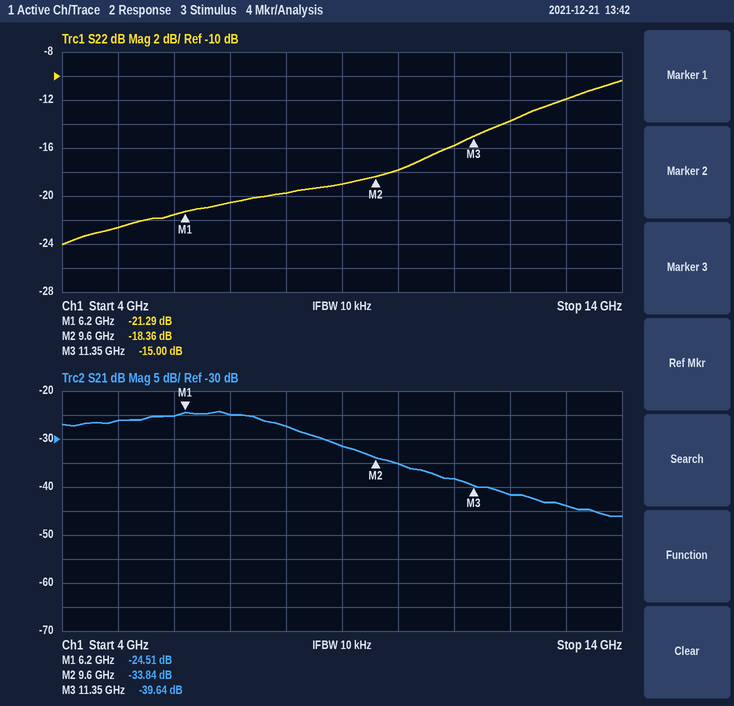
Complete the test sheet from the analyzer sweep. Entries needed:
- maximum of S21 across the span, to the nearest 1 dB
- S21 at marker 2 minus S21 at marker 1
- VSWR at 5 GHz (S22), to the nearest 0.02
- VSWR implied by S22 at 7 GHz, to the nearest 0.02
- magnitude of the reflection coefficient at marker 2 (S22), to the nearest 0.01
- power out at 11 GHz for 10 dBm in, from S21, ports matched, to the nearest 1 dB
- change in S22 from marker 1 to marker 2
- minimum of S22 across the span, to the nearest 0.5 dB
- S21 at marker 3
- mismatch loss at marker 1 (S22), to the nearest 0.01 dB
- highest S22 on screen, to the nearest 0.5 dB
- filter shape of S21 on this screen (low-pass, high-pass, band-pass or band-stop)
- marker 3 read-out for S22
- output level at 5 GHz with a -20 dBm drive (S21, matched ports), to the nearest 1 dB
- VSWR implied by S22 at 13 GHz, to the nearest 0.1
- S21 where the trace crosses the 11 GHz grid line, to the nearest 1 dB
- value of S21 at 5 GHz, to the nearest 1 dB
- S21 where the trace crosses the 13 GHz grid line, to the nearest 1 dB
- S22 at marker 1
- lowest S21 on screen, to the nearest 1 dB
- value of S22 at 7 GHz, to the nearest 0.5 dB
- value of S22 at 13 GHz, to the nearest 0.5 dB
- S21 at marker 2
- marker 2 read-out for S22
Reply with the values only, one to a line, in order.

-24 dB
-9.33 dB
1.16
1.20
0.12
-28 dBm
2.93 dB
-24.0 dB
-39.64 dB
0.03 dB
-10.5 dB
low-pass
-15.00 dB
-46 dBm
1.7
-38 dB
-26 dB
-44 dB
-21.29 dB
-46 dB
-20.5 dB
-12.0 dB
-33.84 dB
-18.36 dB
